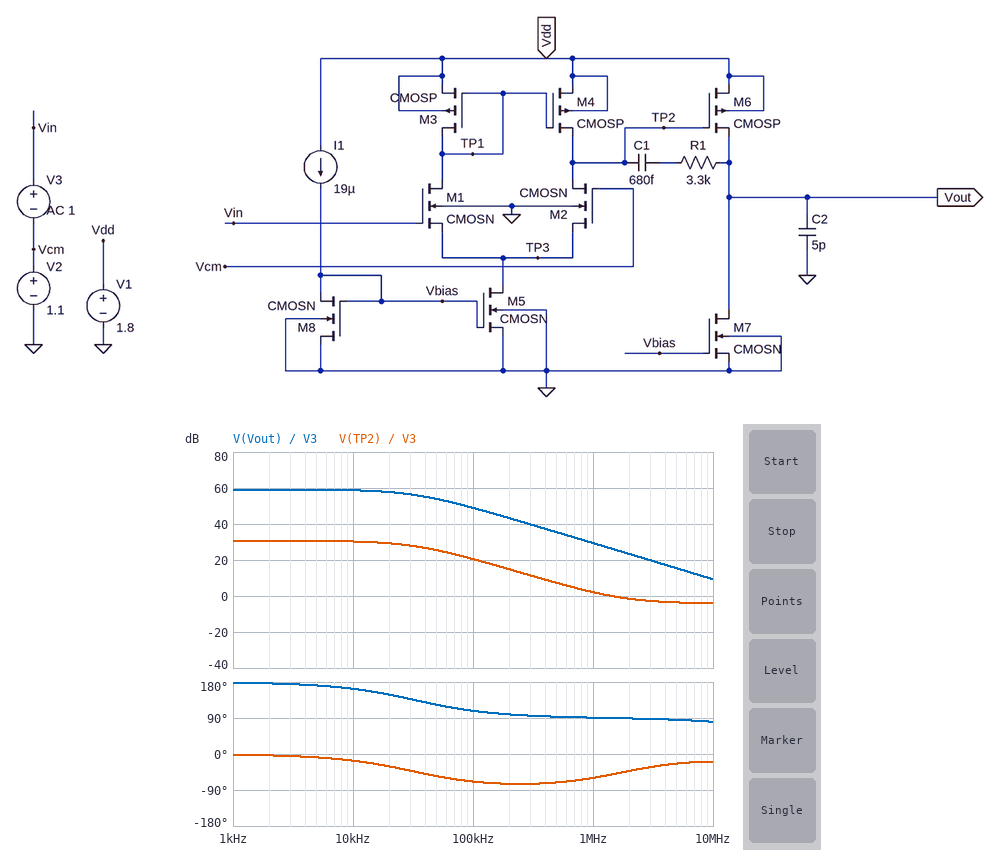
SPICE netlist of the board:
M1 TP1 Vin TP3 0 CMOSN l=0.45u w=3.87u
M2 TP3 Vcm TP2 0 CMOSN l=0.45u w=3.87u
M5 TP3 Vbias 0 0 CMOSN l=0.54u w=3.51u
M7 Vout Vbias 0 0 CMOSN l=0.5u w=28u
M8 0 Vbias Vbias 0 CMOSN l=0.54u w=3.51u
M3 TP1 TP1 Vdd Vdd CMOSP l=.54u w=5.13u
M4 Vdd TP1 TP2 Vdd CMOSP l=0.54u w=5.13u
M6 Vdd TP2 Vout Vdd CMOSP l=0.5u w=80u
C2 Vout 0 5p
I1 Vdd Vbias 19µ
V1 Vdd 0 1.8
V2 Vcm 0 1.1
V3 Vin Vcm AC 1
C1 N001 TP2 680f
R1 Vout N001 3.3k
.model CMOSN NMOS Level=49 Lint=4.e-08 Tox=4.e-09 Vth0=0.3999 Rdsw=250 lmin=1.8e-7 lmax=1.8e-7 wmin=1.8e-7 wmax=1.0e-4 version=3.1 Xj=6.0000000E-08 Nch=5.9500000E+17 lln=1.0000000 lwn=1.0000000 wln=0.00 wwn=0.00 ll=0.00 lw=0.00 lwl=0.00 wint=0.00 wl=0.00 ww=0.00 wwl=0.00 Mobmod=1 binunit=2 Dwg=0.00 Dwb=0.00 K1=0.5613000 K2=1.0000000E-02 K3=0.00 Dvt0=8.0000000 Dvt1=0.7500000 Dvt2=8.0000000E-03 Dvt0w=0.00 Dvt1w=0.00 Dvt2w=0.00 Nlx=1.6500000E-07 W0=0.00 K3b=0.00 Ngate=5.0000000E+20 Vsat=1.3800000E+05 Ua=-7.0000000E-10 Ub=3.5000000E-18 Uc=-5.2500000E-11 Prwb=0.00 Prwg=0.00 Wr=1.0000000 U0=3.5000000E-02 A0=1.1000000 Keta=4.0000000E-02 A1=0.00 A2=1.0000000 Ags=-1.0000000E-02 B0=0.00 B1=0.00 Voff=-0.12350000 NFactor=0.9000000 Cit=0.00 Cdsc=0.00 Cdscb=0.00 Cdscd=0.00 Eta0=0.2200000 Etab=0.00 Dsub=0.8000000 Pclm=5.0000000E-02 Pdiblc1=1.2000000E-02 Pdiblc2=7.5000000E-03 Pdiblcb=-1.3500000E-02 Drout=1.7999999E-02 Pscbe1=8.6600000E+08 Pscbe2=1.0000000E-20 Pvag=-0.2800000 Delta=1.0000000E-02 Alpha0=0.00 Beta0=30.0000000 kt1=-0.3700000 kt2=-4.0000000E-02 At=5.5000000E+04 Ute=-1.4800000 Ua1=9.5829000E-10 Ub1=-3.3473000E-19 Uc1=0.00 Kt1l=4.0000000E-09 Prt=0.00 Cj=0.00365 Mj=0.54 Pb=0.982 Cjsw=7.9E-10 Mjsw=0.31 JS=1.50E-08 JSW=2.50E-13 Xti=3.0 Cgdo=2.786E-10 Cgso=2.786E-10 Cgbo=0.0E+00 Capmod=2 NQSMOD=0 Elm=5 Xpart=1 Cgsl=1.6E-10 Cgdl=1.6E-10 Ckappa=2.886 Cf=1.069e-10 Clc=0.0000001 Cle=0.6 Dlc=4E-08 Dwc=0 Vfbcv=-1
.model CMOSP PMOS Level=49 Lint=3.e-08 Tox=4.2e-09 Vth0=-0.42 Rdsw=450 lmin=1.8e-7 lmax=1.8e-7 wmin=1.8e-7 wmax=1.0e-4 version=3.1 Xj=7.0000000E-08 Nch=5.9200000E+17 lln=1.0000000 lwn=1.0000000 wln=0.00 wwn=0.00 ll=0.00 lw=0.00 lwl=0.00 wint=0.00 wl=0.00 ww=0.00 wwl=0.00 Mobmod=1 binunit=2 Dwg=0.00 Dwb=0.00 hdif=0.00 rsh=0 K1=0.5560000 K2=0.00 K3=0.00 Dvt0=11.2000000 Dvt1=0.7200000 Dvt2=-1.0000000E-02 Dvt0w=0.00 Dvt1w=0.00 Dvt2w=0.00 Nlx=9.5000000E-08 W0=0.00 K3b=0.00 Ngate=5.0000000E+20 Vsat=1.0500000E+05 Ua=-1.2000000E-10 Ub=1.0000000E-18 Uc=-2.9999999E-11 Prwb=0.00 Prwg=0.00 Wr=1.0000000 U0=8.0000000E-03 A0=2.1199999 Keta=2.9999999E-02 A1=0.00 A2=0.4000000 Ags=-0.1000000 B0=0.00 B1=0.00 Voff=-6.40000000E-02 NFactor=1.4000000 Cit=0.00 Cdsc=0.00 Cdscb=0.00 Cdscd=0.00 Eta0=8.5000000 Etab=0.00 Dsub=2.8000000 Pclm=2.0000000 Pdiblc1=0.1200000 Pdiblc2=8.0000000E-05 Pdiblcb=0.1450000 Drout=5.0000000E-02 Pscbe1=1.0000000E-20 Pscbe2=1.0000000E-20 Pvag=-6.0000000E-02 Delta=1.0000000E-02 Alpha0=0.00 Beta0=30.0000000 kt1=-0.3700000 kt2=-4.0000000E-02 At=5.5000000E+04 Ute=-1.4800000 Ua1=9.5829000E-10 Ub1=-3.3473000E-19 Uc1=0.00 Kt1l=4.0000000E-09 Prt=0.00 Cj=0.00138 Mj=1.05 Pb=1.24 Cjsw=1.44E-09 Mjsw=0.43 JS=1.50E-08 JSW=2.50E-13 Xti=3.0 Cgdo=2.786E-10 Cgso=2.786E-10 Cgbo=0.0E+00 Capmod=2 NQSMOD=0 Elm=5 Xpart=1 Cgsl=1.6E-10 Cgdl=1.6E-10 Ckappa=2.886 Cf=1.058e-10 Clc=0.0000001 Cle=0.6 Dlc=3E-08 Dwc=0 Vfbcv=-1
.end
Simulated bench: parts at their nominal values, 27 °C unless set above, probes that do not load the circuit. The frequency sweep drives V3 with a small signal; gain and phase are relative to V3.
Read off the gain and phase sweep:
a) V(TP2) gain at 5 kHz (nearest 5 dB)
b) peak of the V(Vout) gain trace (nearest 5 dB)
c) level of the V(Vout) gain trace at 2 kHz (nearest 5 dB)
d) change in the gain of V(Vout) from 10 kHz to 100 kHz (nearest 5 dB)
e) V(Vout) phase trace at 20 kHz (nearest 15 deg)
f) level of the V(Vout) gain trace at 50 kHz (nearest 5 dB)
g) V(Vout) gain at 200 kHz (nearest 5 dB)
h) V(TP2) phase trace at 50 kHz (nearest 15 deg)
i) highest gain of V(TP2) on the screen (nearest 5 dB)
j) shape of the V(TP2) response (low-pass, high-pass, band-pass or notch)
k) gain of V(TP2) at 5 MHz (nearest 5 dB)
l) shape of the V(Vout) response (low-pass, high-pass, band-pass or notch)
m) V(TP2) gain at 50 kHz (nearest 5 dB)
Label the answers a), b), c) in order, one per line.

a) 30 dB
b) 60 dB
c) 60 dB
d) -10 dB
e) 150 deg
f) 55 dB
g) 45 dB
h) -60 deg
i) 30 dB
j) low-pass
k) -5 dB
l) low-pass
m) 25 dB
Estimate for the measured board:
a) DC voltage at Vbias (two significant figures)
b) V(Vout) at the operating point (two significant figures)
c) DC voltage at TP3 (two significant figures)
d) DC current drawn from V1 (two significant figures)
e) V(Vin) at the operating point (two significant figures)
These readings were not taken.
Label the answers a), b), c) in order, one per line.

a) 610 mV
b) 930 mV
c) 430 mV
d) 200 µA
e) 1.1 V
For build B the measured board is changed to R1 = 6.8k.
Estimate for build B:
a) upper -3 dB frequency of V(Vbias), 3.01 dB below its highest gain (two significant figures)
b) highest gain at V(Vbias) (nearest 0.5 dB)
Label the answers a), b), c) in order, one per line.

a) 130 MHz
b) -37.0 dB
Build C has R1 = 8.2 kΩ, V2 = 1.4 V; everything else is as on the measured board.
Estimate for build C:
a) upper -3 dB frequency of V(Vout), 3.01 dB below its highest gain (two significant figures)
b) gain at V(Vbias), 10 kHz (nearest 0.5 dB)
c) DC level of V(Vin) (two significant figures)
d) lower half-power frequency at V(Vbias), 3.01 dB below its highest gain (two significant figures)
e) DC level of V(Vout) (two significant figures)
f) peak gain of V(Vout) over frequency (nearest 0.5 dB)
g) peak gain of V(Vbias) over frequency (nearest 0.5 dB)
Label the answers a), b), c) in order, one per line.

a) 35 kHz
b) -49.5 dB
c) 1.4 V
d) 82 kHz
e) 1.0 V
f) 58.5 dB
g) -36.0 dB
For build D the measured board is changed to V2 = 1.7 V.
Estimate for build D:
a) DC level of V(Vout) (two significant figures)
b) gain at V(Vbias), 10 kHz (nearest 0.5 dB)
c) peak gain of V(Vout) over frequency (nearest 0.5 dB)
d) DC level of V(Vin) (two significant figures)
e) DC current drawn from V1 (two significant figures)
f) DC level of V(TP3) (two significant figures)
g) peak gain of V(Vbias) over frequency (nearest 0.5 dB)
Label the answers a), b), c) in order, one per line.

a) 1.1 V
b) -51.0 dB
c) 57.0 dB
d) 1.7 V
e) 210 µA
f) 900 mV
g) -38.5 dB
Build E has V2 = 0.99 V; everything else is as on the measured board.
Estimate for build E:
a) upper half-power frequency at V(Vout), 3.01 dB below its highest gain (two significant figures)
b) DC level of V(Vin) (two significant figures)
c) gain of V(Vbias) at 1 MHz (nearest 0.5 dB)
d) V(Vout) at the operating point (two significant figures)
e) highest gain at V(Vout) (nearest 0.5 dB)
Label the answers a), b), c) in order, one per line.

a) 32 kHz
b) 990 mV
c) -38.5 dB
d) 890 mV
e) 59.5 dB
